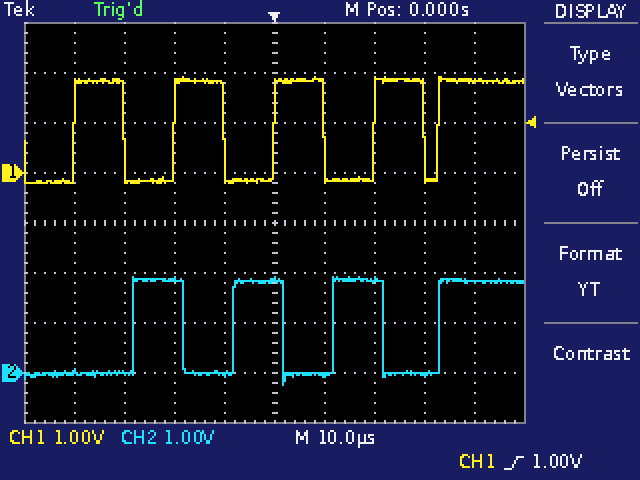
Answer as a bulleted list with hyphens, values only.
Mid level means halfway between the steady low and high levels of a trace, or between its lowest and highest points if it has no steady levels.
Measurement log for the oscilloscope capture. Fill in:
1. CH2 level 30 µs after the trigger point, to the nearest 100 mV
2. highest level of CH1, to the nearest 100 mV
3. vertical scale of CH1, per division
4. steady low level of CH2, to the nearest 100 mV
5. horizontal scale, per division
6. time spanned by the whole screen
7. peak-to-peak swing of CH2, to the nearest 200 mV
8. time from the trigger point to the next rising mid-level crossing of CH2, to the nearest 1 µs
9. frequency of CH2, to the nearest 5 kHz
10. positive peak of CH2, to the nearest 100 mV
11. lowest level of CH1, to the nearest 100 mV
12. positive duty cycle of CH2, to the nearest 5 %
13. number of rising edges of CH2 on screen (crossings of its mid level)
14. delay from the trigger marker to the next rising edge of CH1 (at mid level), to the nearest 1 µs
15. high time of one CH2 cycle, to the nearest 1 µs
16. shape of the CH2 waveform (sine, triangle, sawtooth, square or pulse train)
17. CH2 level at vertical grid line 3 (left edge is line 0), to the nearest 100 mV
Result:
- 0.0 V
- 1.9 V
- 1 V
- 0.0 V
- 10 µs
- 100 µs
- 2.2 V
- 12 µs
- 50 kHz
- 1.9 V
- -200 mV
- 50 %
- 4
- 20 µs
- 10 µs
- square
- 1.9 V
